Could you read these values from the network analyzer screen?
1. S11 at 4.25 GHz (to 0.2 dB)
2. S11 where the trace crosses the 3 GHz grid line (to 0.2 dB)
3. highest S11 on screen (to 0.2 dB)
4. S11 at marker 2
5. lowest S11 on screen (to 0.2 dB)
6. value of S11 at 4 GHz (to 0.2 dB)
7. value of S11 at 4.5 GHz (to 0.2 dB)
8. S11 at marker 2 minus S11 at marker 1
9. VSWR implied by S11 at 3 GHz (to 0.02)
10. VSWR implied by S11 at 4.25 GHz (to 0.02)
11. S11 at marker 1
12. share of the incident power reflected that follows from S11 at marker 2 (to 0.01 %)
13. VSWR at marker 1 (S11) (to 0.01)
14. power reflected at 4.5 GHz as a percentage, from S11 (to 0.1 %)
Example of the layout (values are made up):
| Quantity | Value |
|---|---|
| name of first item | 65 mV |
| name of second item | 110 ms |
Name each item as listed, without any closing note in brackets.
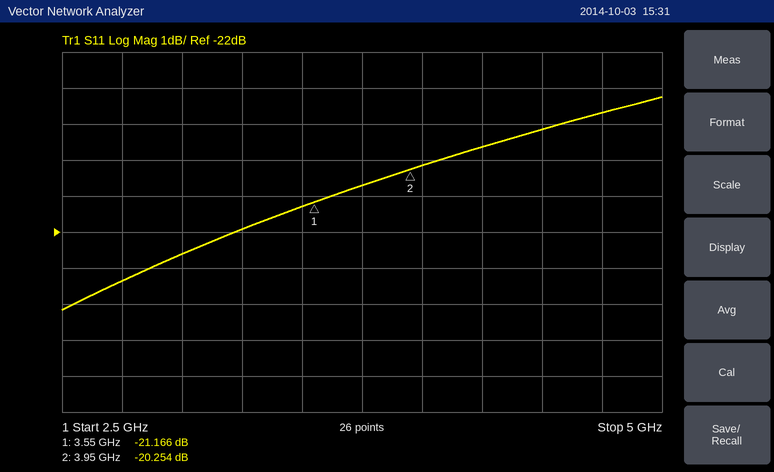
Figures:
| Quantity | Value |
|---|---|
| S11 at 4.25 GHz | -19.6 dB |
| S11 where the trace crosses the 3 GHz grid line | -22.6 dB |
| highest S11 on screen | -18.2 dB |
| S11 at marker 2 | -20.254 dB |
| lowest S11 on screen | -24.2 dB |
| value of S11 at 4 GHz | -20.2 dB |
| value of S11 at 4.5 GHz | -19.2 dB |
| S11 at marker 2 minus S11 at marker 1 | 0.912 dB |
| VSWR implied by S11 at 3 GHz | 1.16 |
| VSWR implied by S11 at 4.25 GHz | 1.24 |
| S11 at marker 1 | -21.166 dB |
| share of the incident power reflected that follows from S11 at marker 2 | 0.94 % |
| VSWR at marker 1 (S11) | 1.19 |
| power reflected at 4.5 GHz as a percentage, from S11 | 1.2 % |
